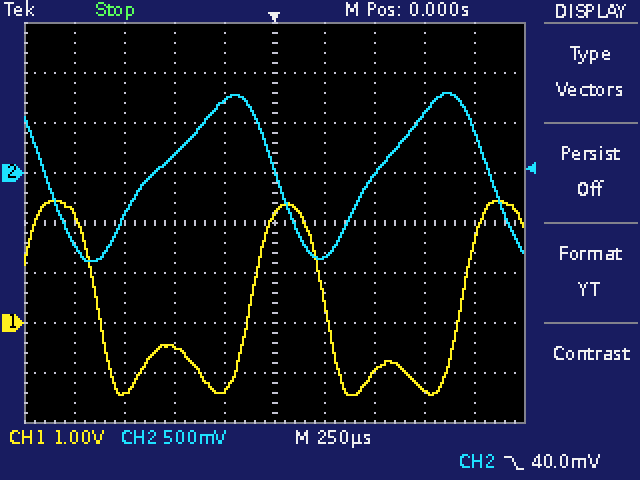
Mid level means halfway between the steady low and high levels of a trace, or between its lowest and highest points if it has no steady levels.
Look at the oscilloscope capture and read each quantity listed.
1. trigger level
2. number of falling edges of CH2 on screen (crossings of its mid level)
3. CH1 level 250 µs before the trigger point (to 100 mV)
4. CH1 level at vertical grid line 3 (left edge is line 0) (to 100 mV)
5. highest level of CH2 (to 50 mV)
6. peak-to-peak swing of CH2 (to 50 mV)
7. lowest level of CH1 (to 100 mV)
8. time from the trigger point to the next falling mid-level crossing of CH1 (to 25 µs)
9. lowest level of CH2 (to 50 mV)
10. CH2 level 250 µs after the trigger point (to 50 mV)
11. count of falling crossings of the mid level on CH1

40.0 mV
3
-1.3 V
-500 mV
800 mV
1.70 V
-1.4 V
250 µs
-900 mV
-850 mV
2
